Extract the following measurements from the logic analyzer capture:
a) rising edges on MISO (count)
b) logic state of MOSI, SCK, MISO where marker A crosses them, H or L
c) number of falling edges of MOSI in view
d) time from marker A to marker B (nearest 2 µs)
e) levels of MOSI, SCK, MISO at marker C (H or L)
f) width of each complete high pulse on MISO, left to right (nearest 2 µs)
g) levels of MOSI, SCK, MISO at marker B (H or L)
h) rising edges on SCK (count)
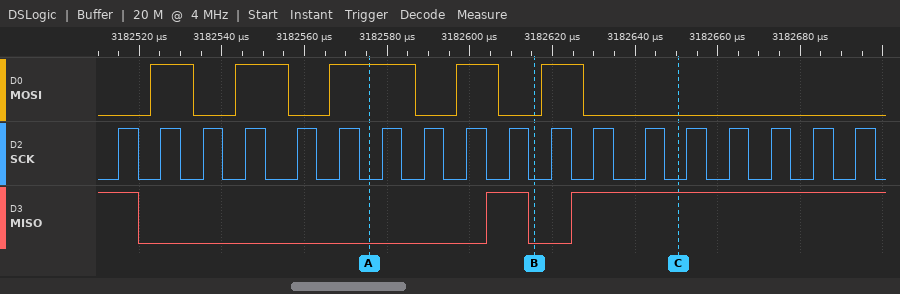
2
MOSI=H, SCK=L, MISO=L
5
40 µs
MOSI=L, SCK=L, MISO=H
10 µs
MOSI=L, SCK=L, MISO=L
18
